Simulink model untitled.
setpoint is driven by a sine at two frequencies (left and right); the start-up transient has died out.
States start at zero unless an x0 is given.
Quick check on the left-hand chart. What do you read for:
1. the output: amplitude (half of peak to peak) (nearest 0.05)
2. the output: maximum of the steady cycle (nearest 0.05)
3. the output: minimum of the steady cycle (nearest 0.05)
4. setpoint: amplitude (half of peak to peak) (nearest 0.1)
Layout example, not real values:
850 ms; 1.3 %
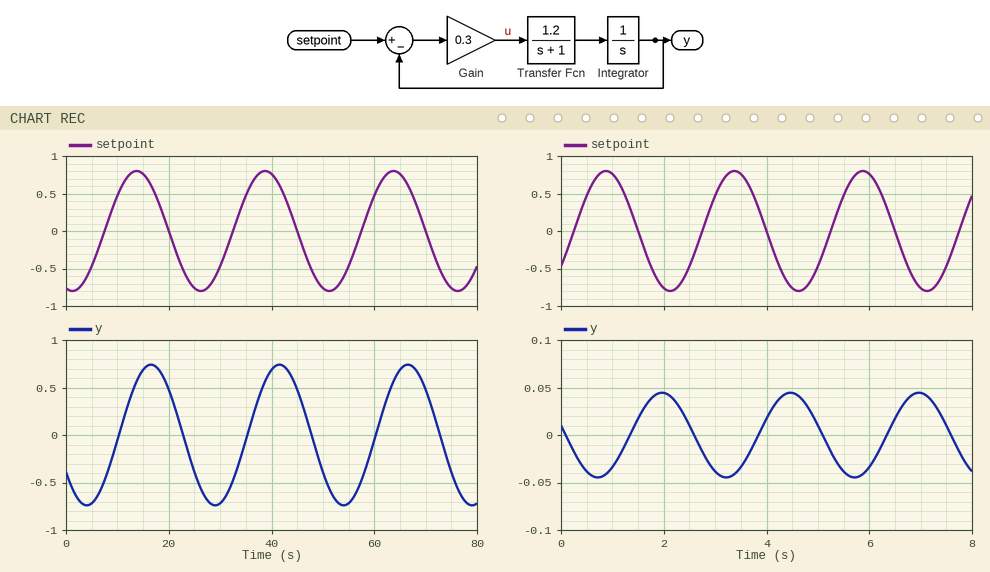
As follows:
0.75; 0.75; -0.75; 0.8
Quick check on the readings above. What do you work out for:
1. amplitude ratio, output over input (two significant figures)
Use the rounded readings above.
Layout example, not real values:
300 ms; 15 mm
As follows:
0.94
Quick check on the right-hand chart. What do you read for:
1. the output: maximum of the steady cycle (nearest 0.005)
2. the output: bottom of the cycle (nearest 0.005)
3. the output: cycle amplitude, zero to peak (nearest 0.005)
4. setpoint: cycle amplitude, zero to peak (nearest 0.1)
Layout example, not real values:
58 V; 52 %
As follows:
0.045; -0.045; 0.045; 0.8
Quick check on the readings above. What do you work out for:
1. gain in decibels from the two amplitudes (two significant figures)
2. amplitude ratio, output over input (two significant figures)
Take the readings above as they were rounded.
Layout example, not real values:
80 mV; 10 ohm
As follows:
-25 dB; 0.056
